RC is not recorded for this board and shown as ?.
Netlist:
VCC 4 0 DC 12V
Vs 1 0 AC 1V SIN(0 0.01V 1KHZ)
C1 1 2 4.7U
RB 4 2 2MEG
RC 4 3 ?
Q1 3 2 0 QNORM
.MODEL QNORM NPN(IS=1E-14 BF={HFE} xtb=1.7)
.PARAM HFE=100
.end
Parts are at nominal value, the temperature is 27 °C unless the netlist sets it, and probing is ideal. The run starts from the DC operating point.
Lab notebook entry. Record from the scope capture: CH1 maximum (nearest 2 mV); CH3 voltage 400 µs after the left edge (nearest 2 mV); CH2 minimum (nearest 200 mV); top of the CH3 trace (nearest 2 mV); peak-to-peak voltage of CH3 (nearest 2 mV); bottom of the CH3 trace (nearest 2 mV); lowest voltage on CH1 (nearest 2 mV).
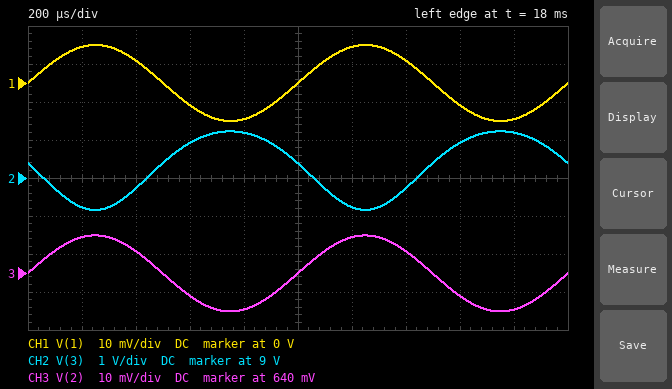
10 mV
646 mV
8.2 V
650 mV
20 mV
630 mV
-10 mV
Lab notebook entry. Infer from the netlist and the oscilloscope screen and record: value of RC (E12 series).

4.7 kΩ
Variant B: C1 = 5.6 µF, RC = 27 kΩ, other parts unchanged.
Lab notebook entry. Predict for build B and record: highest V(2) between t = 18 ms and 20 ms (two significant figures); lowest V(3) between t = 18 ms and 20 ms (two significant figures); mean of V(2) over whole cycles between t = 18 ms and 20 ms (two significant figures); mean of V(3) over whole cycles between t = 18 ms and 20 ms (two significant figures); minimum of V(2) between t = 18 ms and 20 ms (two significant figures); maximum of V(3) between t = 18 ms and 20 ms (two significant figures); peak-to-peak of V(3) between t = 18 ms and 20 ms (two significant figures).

640 mV
86 mV
630 mV
3.1 V
620 mV
6.1 V
6.0 V
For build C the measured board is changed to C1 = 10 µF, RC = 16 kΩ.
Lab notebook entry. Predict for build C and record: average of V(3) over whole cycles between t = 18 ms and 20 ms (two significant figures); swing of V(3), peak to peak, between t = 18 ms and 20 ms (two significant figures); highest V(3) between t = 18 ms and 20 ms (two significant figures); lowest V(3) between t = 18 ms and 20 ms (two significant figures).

3.5 V
6.3 V
6.4 V
120 mV
